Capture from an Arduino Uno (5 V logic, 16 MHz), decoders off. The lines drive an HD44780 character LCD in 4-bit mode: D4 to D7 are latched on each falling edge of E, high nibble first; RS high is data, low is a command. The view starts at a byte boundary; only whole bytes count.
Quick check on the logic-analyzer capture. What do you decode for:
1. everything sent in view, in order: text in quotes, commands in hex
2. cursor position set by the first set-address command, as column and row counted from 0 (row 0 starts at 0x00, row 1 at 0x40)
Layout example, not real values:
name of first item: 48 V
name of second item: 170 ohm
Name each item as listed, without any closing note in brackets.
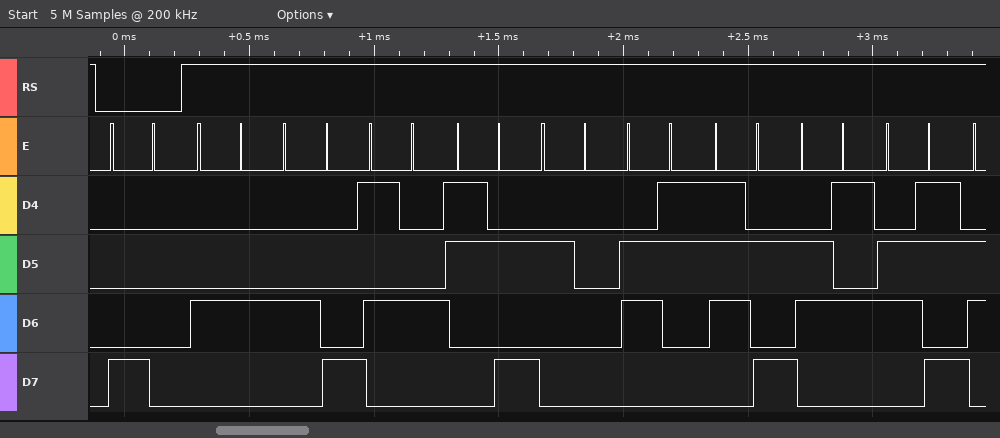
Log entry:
everything sent in view, in order: text in quotes, commands in hex: 0x80 "DHT: czek"
cursor position set by the first set-address command, as column and row counted from 0: column 0, row 0
